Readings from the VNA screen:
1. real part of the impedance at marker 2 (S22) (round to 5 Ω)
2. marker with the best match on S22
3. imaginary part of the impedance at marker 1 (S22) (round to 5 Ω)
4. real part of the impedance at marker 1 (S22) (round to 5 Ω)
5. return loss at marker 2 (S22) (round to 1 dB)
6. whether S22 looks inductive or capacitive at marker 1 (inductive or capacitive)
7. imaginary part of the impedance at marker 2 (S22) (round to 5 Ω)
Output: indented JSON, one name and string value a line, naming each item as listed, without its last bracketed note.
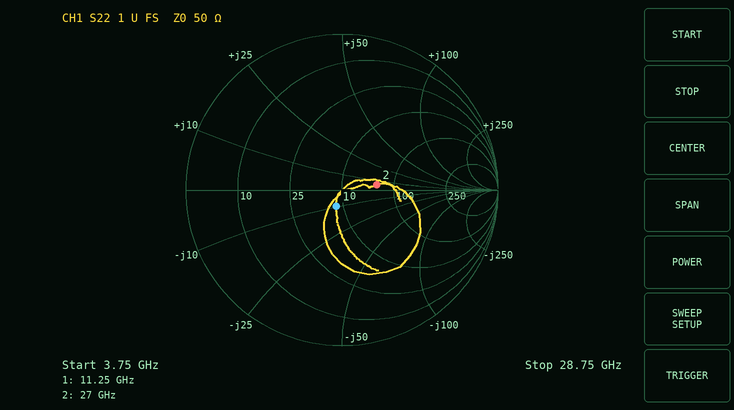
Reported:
{
  "real part of the impedance at marker 2 (S22)": "80 Ω",
  "marker with the best match on S22": "marker 1",
  "imaginary part of the impedance at marker 1 (S22)": "-10 Ω",
  "real part of the impedance at marker 1 (S22)": "45 Ω",
  "return loss at marker 2 (S22)": "13 dB",
  "whether S22 looks inductive or capacitive at marker 1": "capacitive",
  "imaginary part of the impedance at marker 2 (S22)": "+5 Ω"
}
